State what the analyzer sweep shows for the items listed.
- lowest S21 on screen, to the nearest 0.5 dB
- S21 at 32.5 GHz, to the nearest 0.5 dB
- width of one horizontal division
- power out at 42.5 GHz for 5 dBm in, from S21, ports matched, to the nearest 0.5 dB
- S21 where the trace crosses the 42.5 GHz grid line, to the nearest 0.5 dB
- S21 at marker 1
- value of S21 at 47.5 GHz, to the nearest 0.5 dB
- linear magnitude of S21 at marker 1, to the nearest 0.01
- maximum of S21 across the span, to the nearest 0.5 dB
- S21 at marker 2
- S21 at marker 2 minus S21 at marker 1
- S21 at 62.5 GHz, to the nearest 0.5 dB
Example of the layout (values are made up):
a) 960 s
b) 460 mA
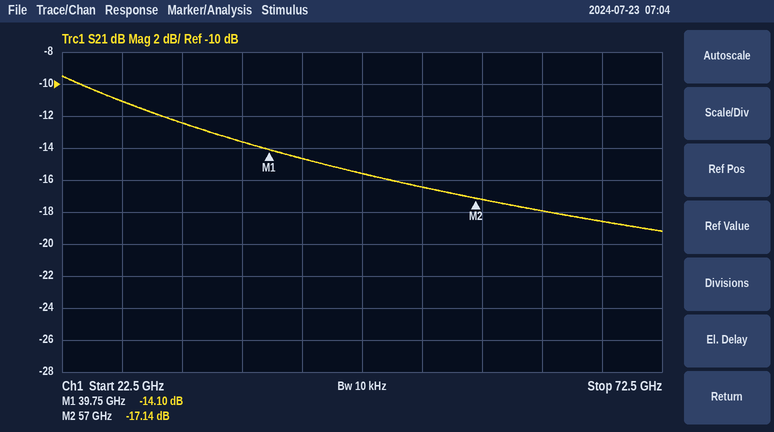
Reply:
a) -19.0 dB
b) -12.5 dB
c) 5 GHz
d) -9.5 dBm
e) -14.5 dB
f) -14.10 dB
g) -15.5 dB
h) 0.20
i) -9.5 dB
j) -17.14 dB
k) -3.04 dB
l) -18.0 dB
